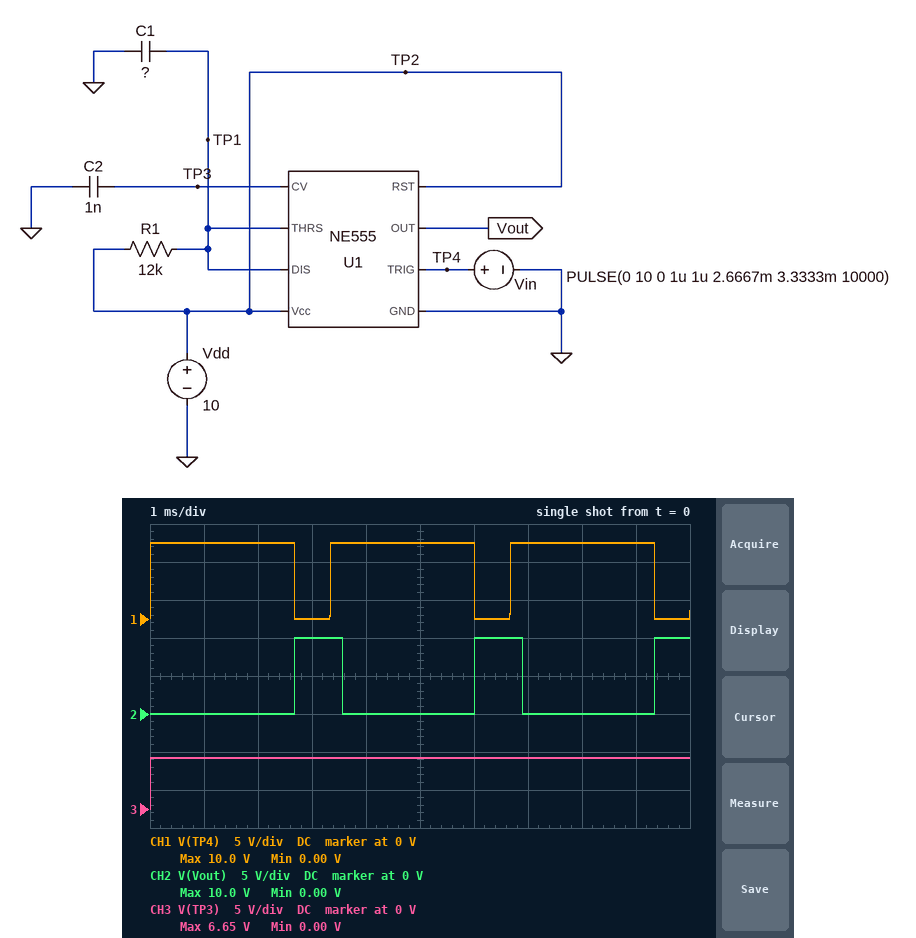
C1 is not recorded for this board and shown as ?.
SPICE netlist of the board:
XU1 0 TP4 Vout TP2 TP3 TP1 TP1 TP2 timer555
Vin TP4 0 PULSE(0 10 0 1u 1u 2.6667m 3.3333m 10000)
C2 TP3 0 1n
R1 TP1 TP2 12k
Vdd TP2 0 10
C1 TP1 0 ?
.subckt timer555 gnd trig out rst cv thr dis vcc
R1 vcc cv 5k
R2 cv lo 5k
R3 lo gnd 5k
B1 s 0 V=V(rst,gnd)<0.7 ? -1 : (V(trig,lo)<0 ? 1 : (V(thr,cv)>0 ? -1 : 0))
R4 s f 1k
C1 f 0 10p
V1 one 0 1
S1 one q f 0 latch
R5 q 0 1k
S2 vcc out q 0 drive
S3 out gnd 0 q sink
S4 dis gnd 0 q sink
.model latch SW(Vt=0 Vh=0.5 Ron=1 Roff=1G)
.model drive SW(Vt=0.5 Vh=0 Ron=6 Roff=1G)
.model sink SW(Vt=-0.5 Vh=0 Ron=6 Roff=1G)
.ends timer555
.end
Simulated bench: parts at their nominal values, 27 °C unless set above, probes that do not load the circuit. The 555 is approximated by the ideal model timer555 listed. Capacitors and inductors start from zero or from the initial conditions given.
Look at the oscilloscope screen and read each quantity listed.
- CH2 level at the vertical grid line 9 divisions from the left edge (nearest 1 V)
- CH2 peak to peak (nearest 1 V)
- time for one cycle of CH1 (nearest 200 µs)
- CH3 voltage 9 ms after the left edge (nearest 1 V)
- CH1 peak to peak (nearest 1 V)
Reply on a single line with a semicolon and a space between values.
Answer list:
0 V; 10 V; 3.4 ms; 7 V; 10 V
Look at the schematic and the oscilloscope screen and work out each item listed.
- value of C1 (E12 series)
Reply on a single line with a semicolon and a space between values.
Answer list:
68 nF
